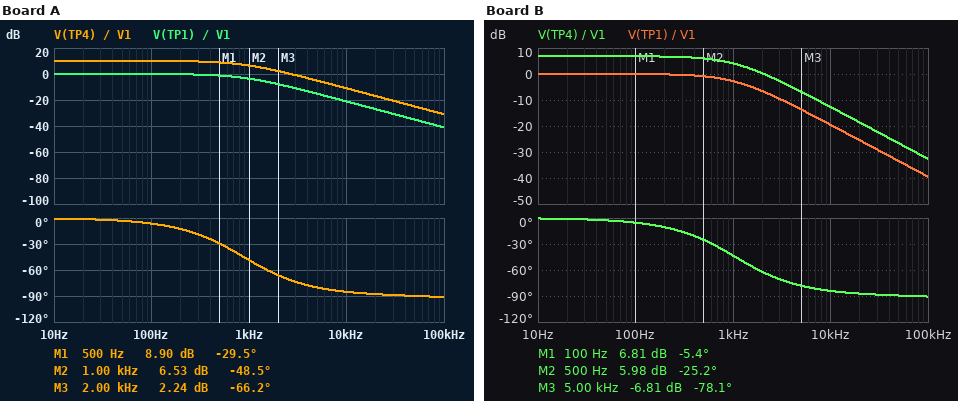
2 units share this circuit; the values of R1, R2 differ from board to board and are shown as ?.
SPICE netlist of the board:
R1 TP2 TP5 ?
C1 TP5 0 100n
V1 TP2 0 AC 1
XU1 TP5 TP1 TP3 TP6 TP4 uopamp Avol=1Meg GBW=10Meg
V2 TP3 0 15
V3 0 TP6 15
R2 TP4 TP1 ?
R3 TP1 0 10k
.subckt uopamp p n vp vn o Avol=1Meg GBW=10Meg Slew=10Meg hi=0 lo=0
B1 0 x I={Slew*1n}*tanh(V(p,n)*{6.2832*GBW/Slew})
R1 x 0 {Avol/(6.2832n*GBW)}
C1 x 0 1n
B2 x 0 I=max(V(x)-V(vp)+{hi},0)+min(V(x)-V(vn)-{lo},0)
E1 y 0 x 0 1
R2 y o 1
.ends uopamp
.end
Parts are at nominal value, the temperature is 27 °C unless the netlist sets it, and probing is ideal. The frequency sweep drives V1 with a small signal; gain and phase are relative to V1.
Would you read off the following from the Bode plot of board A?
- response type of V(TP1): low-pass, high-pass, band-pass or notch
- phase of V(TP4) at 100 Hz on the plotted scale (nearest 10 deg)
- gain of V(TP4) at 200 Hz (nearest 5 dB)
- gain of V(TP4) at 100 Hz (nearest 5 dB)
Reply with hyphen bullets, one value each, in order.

- low-pass
- -10 deg
- 10 dB
- 10 dB
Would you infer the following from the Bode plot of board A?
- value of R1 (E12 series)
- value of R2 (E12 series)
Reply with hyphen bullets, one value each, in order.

- 1.8 kΩ
- 22 kΩ
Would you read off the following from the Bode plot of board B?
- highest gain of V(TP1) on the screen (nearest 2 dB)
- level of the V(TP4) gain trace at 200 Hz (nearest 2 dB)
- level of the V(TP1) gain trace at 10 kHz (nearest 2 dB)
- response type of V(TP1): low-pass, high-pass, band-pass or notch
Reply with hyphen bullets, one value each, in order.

- 0 dB
- 6 dB
- -20 dB
- low-pass
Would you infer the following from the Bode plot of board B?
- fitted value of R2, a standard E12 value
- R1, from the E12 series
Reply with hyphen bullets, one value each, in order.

- 12 kΩ
- 1.5 kΩ
